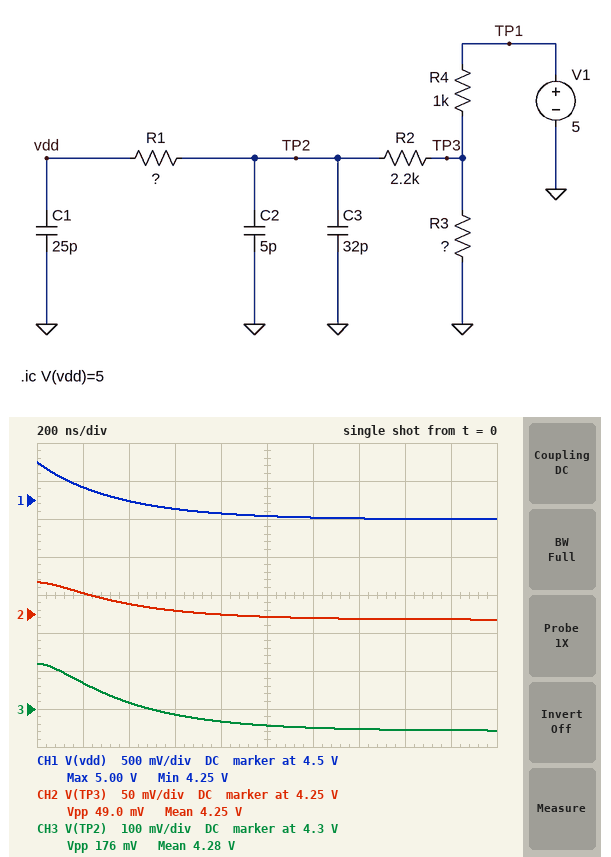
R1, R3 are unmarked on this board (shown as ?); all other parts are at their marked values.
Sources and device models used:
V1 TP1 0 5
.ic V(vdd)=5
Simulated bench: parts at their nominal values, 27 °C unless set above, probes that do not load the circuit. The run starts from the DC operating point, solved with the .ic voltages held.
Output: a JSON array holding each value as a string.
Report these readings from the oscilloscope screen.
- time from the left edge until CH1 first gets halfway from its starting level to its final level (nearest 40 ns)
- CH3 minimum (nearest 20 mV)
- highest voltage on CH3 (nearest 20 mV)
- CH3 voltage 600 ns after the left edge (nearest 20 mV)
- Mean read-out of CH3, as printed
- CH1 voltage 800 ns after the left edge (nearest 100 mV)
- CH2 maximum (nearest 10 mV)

["240 ns", "4.24 V", "4.42 V", "4.28 V", "4.28 V", "4.3 V", "4.29 V"]
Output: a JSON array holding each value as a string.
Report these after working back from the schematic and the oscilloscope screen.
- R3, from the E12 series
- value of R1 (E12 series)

["5.6 kΩ", "10 kΩ"]
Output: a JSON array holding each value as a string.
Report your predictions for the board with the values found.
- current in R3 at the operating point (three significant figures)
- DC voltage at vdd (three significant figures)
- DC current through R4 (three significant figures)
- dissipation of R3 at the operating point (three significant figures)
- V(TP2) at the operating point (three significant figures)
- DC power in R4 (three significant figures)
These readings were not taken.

["758 µA", "4.24 V", "758 µA", "3.21 mW", "4.24 V", "574 µW"]
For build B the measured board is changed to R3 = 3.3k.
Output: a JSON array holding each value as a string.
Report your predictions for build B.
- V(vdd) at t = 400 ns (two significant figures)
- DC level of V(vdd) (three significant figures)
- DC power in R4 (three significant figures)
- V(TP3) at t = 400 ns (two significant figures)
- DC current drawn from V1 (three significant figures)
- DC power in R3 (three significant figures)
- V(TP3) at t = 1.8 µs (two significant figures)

["4.2 V", "3.84 V", "1.35 mW", "3.9 V", "1.16 mA", "4.46 mW", "3.8 V"]
